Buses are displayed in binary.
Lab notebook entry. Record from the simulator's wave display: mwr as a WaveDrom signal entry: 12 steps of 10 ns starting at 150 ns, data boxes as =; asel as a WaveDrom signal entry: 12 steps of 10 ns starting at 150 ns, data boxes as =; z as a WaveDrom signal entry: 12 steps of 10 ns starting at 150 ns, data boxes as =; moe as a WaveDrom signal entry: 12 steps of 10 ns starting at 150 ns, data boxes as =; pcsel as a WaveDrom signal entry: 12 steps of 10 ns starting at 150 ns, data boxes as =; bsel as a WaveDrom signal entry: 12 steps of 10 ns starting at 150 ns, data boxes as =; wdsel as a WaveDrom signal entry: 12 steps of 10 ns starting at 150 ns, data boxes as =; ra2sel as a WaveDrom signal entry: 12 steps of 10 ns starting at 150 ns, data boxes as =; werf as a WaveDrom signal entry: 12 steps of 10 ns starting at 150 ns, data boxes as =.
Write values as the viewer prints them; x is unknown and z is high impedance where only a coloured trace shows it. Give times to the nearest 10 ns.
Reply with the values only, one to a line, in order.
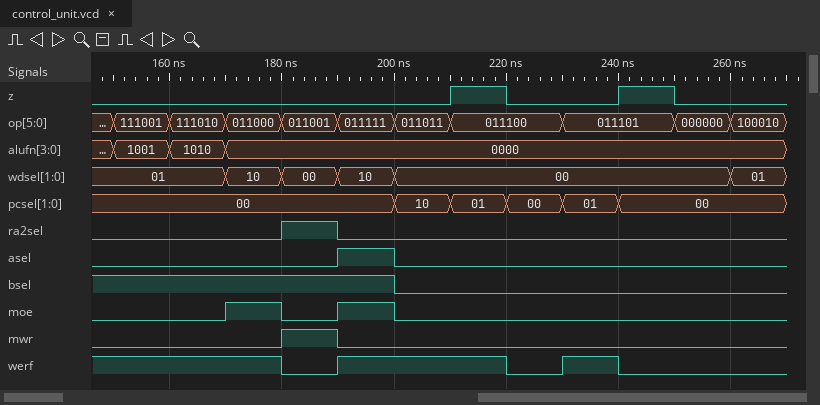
{name: 'mwr', wave: '0..10.......'}
{name: 'asel', wave: '0...10......'}
{name: 'z', wave: '0.....10.10.'}
{name: 'moe', wave: '0.1010......'}
{name: 'pcsel', wave: '=....=====..', data: '00 10 01 00 01 00'}
{name: 'bsel', wave: '1....0......'}
{name: 'wdsel', wave: '=.====.....=', data: '01 10 00 10 00 01'}
{name: 'ra2sel', wave: '0..10.......'}
{name: 'werf', wave: '1..01..010..'}
